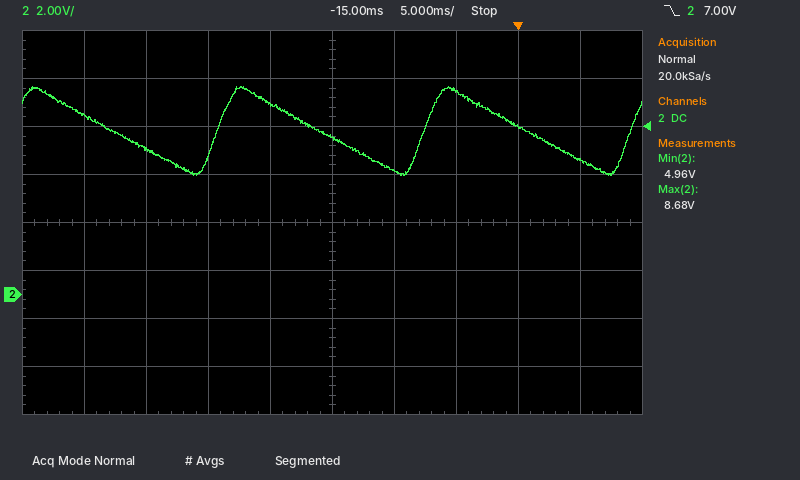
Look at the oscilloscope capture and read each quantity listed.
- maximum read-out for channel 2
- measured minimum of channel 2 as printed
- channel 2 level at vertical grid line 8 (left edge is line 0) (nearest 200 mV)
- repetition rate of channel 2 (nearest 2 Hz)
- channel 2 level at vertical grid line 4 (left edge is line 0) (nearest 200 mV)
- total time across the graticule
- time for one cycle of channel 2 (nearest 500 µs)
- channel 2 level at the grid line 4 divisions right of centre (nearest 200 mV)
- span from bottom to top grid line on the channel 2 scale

8.68 V
4.96 V
7.0 V
60 Hz
8.0 V
50 ms
16.5 ms
5.6 V
16 V
